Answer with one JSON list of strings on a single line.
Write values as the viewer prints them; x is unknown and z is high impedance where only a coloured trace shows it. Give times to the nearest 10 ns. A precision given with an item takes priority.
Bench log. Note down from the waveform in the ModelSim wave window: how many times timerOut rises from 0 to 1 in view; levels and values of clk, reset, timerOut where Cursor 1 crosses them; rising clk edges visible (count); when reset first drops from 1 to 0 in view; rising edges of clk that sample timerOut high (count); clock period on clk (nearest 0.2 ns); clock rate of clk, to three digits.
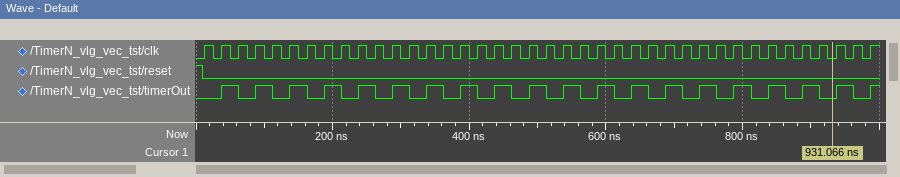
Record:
["20", "clk=0, reset=0, timerOut=0", "40", "10 ns", "19", "25 ns", "40.0 MHz"]
